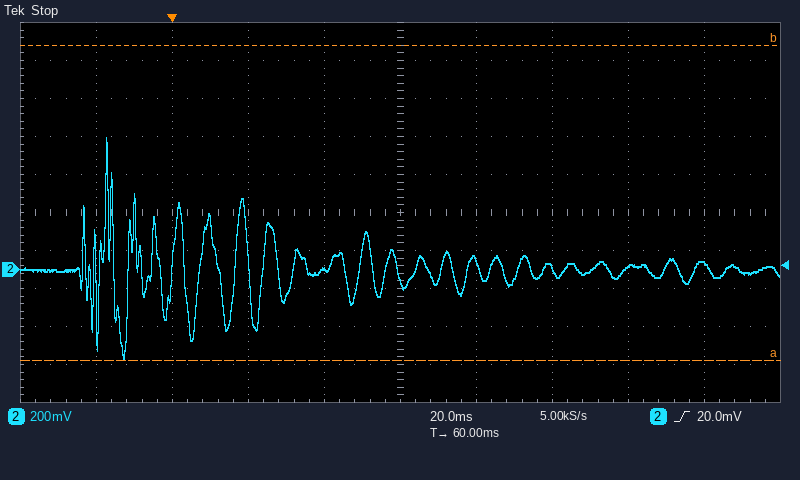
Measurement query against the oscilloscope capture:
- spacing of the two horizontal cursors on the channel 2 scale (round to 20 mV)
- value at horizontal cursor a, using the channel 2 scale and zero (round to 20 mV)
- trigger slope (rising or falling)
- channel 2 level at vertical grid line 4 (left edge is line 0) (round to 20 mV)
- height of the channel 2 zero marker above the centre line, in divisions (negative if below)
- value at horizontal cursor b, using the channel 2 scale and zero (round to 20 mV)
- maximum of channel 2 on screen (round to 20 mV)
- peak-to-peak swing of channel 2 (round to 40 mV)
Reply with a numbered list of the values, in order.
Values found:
1. 1.66 V
2. -480 mV
3. rising
4. 0 mV
5. -1.5 div
6. 1.18 V
7. 700 mV
8. 1.16 V
